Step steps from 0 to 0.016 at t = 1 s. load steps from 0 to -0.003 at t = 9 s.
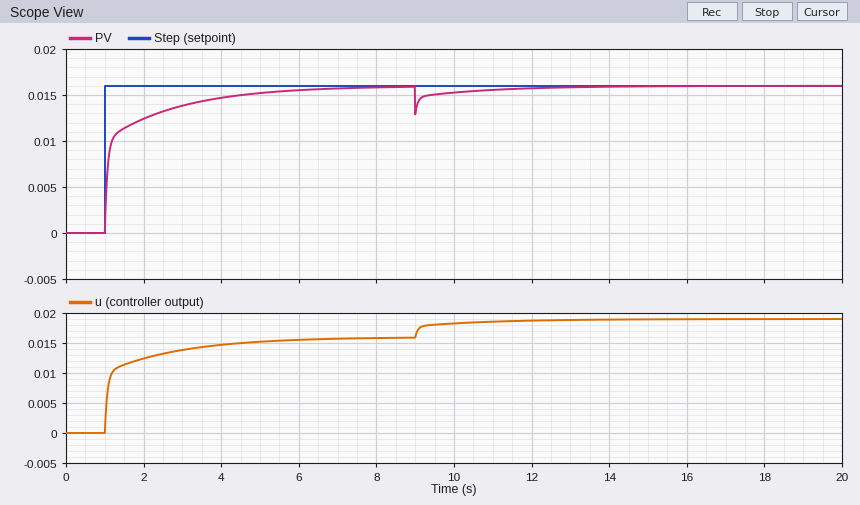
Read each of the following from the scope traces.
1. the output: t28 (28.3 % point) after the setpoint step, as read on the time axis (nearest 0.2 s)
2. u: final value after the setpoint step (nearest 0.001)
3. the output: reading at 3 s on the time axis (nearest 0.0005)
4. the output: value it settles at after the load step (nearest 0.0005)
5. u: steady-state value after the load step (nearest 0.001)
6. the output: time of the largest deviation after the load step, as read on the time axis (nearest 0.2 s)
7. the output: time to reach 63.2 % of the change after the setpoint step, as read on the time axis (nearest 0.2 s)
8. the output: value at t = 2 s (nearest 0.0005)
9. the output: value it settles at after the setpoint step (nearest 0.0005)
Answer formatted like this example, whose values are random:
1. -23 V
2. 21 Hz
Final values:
1. 1.0 s
2. 0.016
3. 0.0140
4. 0.0160
5. 0.019
6. 9.0 s
7. 1.2 s
8. 0.0125
9. 0.0160
